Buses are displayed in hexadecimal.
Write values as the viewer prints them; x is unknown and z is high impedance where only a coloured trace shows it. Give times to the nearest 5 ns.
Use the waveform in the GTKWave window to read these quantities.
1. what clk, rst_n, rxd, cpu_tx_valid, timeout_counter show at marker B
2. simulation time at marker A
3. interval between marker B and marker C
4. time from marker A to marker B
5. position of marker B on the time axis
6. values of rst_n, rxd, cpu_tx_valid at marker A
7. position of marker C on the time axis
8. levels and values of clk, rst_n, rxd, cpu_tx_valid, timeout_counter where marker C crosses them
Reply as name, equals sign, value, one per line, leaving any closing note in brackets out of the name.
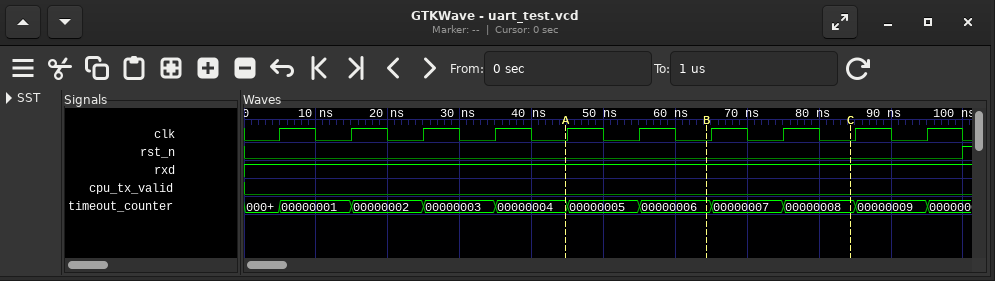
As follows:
what clk, rst_n, rxd, cpu_tx_valid, timeout_counter show at marker B = clk=0, rst_n=0, rxd=1, cpu_tx_valid=0, timeout_counter=00000006
simulation time at marker A = 45 ns
interval between marker B and marker C = 20 ns
time from marker A to marker B = 20 ns
position of marker B on the time axis = 65 ns
values of rst_n, rxd, cpu_tx_valid at marker A = rst_n=0, rxd=1, cpu_tx_valid=0
position of marker C on the time axis = 85 ns
levels and values of clk, rst_n, rxd, cpu_tx_valid, timeout_counter where marker C crosses them = clk=0, rst_n=0, rxd=1, cpu_tx_valid=0, timeout_counter=00000008
